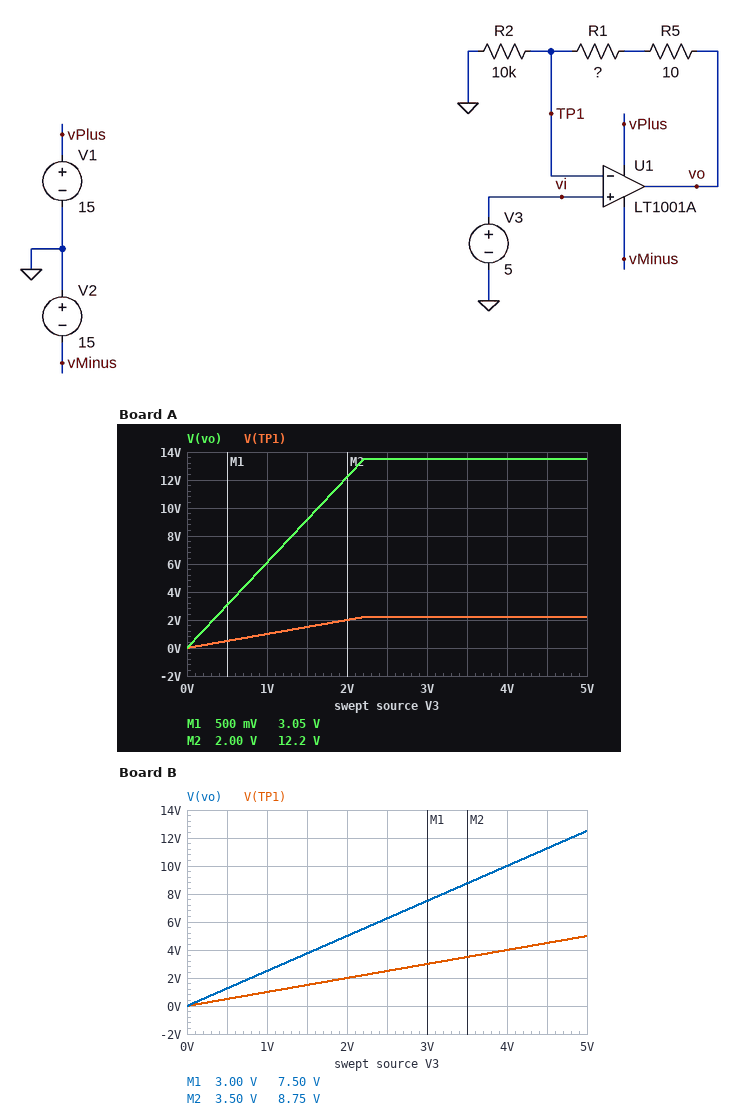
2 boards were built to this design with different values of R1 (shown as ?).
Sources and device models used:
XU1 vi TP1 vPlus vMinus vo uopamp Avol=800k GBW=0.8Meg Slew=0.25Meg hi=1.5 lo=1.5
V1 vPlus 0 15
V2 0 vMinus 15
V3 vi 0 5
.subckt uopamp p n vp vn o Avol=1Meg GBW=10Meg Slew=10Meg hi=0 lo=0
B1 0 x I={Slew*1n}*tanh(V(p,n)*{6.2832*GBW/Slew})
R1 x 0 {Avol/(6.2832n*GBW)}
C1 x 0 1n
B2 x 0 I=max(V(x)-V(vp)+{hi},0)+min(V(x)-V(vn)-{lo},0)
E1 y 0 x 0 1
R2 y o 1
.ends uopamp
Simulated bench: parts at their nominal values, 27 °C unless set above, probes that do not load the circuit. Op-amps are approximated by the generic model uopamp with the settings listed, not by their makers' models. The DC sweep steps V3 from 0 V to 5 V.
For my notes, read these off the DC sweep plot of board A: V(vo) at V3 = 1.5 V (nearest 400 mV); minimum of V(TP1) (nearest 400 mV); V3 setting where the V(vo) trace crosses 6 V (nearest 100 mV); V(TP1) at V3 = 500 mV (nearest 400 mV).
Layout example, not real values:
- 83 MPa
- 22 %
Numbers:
- 9.2 V
- 0 V
- 1.0 V
- 400 mV
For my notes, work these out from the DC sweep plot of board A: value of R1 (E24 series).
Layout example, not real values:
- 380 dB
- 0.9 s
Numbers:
- 51 kΩ
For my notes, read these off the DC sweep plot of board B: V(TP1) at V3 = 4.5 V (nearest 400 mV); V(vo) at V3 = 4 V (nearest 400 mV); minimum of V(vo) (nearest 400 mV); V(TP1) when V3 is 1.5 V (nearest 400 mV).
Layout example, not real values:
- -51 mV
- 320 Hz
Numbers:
- 4.4 V
- 10.0 V
- 0 V
- 1.6 V
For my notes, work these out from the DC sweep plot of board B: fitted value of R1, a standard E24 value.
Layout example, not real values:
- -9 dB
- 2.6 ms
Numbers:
- 15 kΩ
